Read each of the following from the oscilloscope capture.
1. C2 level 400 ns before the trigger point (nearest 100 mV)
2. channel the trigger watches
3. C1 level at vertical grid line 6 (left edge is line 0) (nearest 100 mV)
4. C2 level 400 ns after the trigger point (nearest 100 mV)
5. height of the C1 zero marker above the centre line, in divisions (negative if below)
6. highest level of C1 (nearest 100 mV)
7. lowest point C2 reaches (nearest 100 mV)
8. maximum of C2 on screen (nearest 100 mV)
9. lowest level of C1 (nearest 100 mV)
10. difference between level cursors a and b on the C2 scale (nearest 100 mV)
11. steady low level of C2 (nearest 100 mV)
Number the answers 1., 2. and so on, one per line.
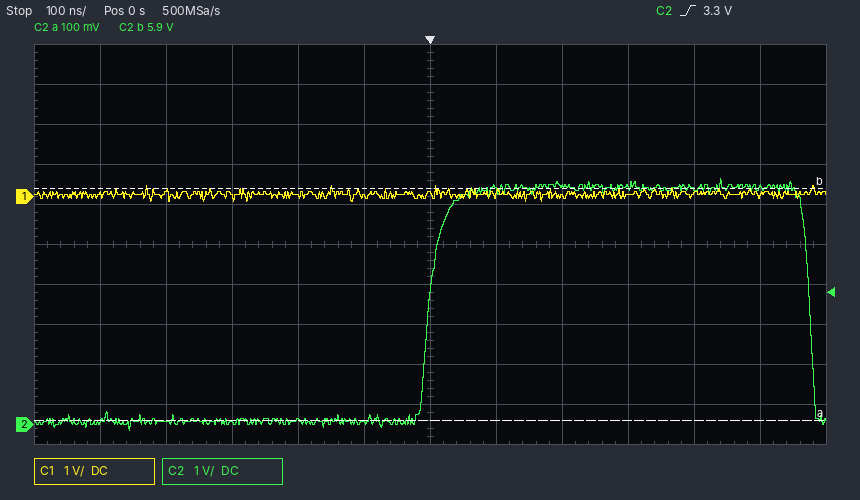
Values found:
1. 100 mV
2. C2
3. 0.0 V
4. 5.9 V
5. +1.2 div
6. 300 mV
7. -200 mV
8. 6.2 V
9. -100 mV
10. 5.8 V
11. 100 mV
